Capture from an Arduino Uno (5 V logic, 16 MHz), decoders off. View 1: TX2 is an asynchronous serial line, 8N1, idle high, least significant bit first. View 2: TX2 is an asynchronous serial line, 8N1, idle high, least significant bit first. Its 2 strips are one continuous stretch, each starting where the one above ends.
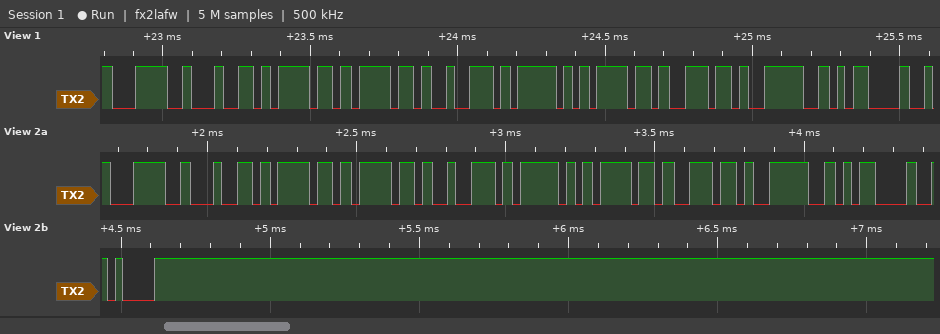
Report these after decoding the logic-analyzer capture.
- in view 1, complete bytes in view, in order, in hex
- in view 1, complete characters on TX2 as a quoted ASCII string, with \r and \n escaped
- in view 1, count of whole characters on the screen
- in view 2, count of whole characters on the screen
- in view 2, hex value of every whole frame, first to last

3C 64 6F 6F 72 5F 6F 6E 3E 0D
"<door_on>\r"
10
11
3C 64 6F 6F 72 5F 6F 6E 3E 0D 0A
